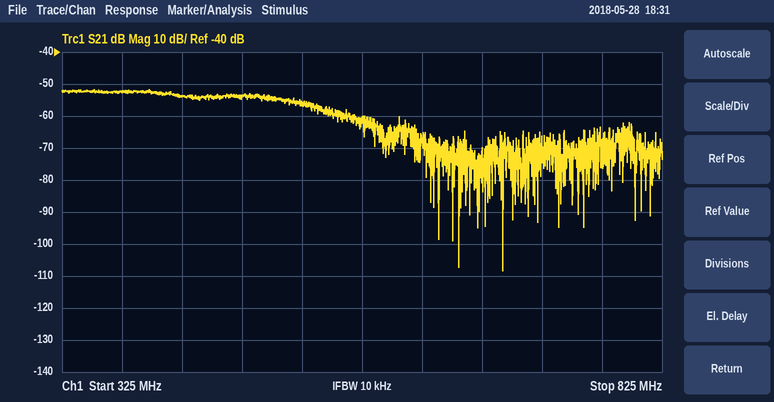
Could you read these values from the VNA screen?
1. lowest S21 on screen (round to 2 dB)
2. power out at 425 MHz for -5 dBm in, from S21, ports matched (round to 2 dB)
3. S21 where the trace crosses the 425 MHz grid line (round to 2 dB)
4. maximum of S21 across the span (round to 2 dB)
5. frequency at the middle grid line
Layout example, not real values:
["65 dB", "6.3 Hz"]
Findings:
["-108 dB", "-58 dBm", "-54 dB", "-52 dB", "575 MHz"]
